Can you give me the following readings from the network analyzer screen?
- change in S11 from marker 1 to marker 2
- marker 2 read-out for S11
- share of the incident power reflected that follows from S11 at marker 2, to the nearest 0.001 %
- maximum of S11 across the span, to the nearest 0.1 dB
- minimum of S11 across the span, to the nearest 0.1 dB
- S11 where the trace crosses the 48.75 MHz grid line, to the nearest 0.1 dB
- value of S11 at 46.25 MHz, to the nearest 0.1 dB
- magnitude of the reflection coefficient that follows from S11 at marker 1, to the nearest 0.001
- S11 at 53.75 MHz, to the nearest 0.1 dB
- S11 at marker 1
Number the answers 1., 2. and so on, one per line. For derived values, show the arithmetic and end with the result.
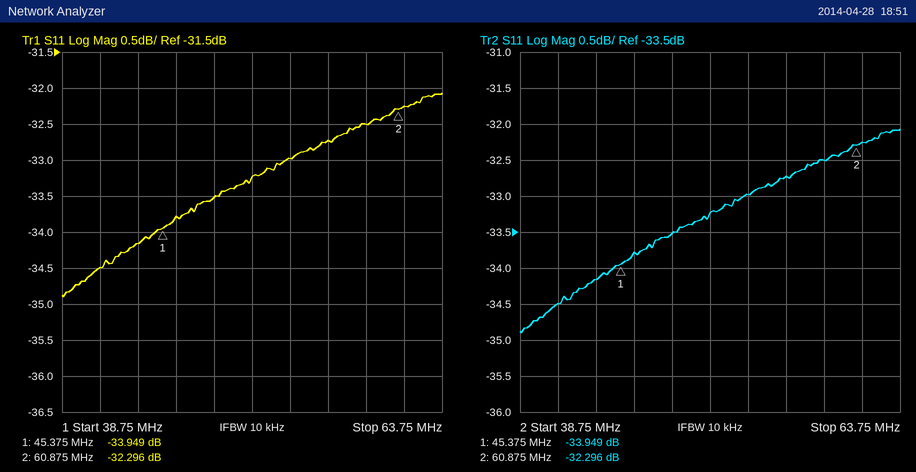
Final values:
1. -32.296 − (-33.949) = 1.653 dB
2. -32.296 dB
3. 10^(-32.296/10) ≈ 0.059 %
4. -32.1 dB
5. -34.9 dB
6. -33.5 dB
7. -33.8 dB
8. 10^(-33.949/20) ≈ 0.020
9. -33.0 dB
10. -33.949 dB
